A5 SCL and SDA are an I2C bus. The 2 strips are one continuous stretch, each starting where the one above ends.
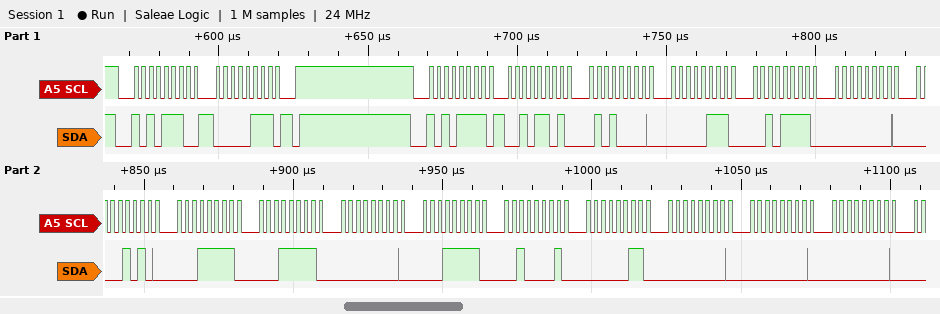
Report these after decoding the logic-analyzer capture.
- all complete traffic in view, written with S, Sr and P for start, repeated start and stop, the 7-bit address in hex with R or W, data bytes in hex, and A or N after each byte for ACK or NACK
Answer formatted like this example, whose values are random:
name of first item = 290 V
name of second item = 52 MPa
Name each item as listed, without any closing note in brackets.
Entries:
all complete traffic in view, written with S, Sr and P for start, repeated start and stop, the 7-bit address in hex with R or W, data bytes in hex, and A or N after each byte for ACK or NACK = S 57W A 07 A P S 57R A 2D A 50 A 07 A 2F A 00 A 0A A 1F A 1F A 00 A 1F A 21 A 03 A 00 A 00 A 00 A
